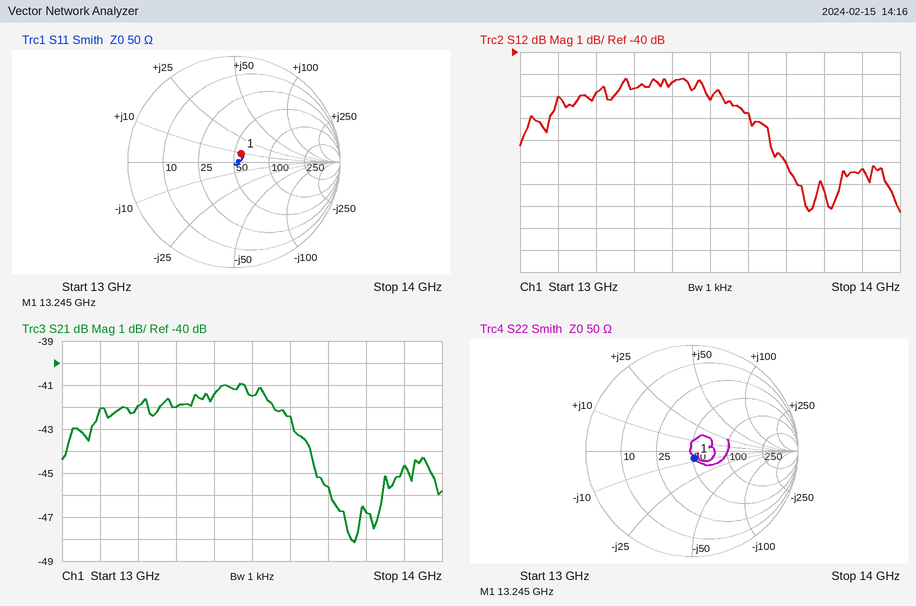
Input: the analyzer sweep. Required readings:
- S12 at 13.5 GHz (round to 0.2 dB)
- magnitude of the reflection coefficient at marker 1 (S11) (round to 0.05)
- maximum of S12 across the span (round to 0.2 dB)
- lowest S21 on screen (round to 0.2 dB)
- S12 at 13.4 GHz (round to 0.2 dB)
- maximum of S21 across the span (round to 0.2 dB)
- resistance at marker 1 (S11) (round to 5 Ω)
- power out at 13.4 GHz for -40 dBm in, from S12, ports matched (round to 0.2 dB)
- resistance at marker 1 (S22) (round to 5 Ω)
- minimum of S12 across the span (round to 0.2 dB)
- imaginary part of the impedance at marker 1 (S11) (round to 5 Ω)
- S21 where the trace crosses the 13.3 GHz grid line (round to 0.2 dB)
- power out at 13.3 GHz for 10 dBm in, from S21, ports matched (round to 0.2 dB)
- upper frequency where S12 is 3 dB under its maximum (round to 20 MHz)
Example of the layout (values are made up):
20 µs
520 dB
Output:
-42.2 dB
0.10
-41.2 dB
-48.2 dB
-41.4 dB
-41.0 dB
55 Ω
-81.4 dBm
50 Ω
-47.2 dB
+10 Ω
-42.0 dB
-32.0 dBm
13.66 GHz
